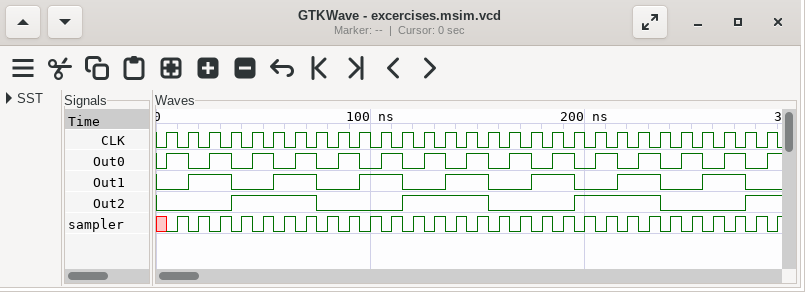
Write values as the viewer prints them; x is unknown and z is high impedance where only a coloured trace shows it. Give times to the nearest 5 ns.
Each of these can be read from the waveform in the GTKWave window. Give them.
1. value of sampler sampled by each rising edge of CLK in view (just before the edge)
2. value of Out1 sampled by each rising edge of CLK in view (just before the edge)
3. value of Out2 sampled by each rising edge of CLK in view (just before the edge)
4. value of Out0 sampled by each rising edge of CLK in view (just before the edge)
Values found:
x 1 1 1 1 1 1 1 1 1 1 1 1 1 1 1 1 1 1 1 1 1 1 1 1 1 1 1 1
0 0 1 1 0 0 1 1 0 0 1 1 0 0 1 1 0 0 1 1 0 0 1 1 0 0 1 1 0
0 0 0 0 1 1 1 1 0 0 0 0 1 1 1 1 0 0 0 0 1 1 1 1 0 0 0 0 1
0 1 0 1 0 1 0 1 0 1 0 1 0 1 0 1 0 1 0 1 0 1 0 1 0 1 0 1 0
